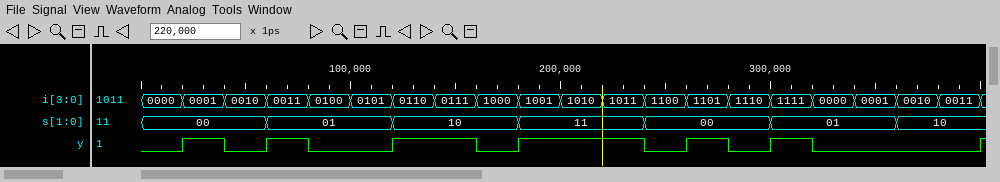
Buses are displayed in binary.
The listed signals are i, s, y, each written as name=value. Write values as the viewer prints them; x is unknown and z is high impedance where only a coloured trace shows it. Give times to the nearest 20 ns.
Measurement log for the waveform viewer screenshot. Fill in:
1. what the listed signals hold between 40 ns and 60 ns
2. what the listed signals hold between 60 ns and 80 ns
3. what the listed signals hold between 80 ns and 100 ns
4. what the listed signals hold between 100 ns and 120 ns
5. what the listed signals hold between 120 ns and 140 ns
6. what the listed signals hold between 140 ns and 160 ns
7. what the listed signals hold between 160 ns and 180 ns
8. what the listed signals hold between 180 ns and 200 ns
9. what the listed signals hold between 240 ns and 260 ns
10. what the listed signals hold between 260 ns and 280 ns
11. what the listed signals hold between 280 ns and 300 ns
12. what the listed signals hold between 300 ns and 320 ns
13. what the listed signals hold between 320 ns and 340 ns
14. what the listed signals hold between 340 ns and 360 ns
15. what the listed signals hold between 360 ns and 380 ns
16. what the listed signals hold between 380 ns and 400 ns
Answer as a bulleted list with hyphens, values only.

- i=0010, s=00, y=0
- i=0011, s=01, y=1
- i=0100, s=01, y=0
- i=0101, s=01, y=0
- i=0110, s=10, y=1
- i=0111, s=10, y=1
- i=1000, s=10, y=0
- i=1001, s=11, y=1
- i=1100, s=00, y=0
- i=1101, s=00, y=1
- i=1110, s=00, y=0
- i=1111, s=01, y=1
- i=0000, s=01, y=0
- i=0001, s=01, y=0
- i=0010, s=10, y=0
- i=0011, s=10, y=0
